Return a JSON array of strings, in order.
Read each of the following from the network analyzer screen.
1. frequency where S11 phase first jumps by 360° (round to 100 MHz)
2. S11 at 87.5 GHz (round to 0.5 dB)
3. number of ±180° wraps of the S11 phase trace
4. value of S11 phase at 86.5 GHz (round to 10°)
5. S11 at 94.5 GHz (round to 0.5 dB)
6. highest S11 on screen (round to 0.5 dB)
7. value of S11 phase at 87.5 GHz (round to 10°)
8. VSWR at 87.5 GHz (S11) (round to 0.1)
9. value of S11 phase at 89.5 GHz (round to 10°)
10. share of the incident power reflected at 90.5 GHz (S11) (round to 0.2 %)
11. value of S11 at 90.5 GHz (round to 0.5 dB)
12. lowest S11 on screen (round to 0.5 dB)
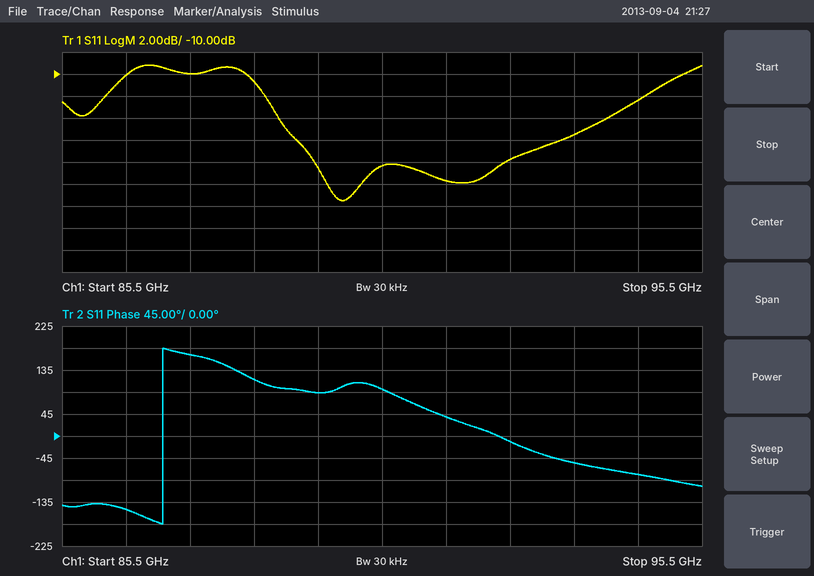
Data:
["87.1 GHz", "-10.0 dB", "1", "-150°", "-12.5 dB", "-9.0 dB", "170°", "1.9", "90°", "1.4 %", "-18.5 dB", "-21.5 dB"]
